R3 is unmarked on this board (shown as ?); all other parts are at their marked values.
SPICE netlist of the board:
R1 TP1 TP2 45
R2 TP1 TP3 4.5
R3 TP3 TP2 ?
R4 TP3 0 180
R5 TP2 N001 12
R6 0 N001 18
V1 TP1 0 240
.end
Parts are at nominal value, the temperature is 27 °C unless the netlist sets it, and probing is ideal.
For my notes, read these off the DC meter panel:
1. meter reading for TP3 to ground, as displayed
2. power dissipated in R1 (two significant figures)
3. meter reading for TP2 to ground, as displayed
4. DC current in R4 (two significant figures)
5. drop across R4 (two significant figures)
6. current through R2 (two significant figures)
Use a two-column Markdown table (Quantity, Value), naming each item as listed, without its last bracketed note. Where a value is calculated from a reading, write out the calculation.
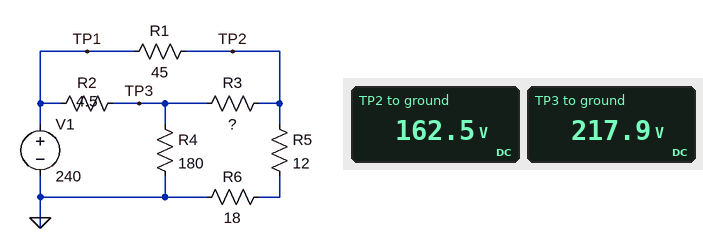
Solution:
| Quantity | Value |
|---|---|
| meter reading for TP3 to ground, as displayed | 217.9 V |
| power dissipated in R1 | (240 V - 162.5 V)^2 / 45 Ω = 130 W |
| meter reading for TP2 to ground, as displayed | 162.5 V |
| DC current in R4 | (217.9 V) / 180 Ω = 1.2 A |
| drop across R4 | 217.9 V = 220 V |
| current through R2 | (240 V - 217.9 V) / 4.5 Ω = 4.9 A |
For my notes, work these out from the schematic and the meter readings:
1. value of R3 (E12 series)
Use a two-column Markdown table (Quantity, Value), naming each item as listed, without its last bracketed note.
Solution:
| Quantity | Value |
|---|---|
| value of R3 | 15 Ω |
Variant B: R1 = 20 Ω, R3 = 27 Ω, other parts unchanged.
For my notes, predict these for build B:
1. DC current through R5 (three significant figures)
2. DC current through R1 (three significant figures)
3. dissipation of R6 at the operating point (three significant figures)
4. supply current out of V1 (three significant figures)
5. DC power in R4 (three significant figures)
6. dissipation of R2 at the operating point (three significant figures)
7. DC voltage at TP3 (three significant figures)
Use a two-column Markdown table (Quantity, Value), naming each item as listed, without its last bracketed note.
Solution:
| Quantity | Value |
|---|---|
| DC current through R5 | 5.63 A |
| DC current through R1 | 3.55 A |
| dissipation of R6 at the operating point | 571 W |
| supply current out of V1 | 6.88 A |
| DC power in R4 | 281 W |
| dissipation of R2 at the operating point | 49.8 W |
| DC voltage at TP3 | 225 V |
